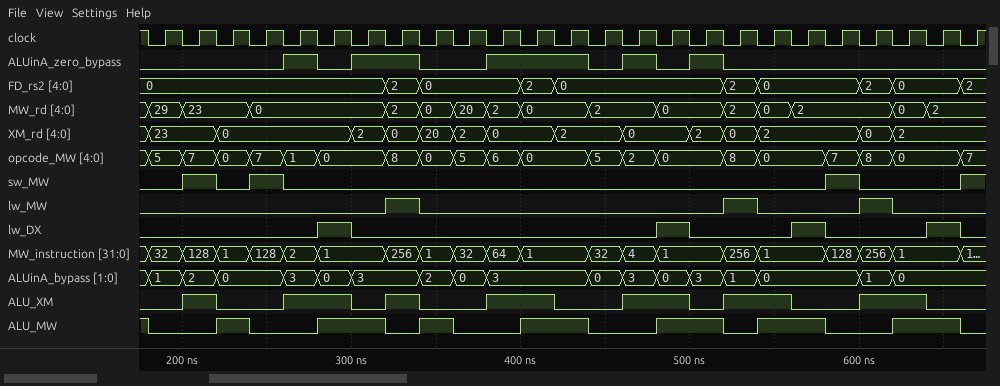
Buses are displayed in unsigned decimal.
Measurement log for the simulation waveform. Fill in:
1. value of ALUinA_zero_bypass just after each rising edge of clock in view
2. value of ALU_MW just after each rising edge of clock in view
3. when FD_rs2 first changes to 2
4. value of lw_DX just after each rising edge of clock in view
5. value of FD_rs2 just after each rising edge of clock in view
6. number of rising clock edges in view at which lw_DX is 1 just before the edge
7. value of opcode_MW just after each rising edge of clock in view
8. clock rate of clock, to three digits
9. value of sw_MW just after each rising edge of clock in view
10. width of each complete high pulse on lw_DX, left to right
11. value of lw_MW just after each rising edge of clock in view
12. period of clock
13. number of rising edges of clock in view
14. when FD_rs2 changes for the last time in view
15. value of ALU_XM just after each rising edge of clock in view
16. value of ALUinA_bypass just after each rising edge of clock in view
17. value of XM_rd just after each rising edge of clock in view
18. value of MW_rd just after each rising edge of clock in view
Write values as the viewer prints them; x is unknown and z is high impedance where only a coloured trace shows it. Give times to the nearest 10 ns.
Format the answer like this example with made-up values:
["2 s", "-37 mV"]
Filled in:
["0 0 0 0 1 0 1 1 0 0 1 1 1 0 1 0 1 0 0 0 0 0 0 0 0", "0 0 1 0 0 1 1 0 1 0 0 1 1 0 0 1 1 0 1 1 0 0 1 1 0", "320 ns", "0 0 0 0 0 1 0 0 0 0 0 0 0 0 0 1 0 0 0 1 0 0 0 1 0", "0, 0, 0, 0, 0, 0, 0, 2, 0, 0, 0, 2, 0, 0, 0, 0, 0, 2, 0, 0, 0, 2, 0, 0, 2", "4", "5, 7, 0, 7, 1, 0, 0, 8, 0, 5, 6, 0, 0, 5, 2, 0, 0, 8, 0, 0, 7, 8, 0, 0, 7", "50.0 MHz", "0 1 0 1 0 0 0 0 0 0 0 0 0 0 0 0 0 0 0 0 1 0 0 0 1", "20 ns, 20 ns, 20 ns, 20 ns", "0 0 0 0 0 0 0 1 0 0 0 0 0 0 0 0 0 1 0 0 0 1 0 0 0", "20 ns", "25", "660 ns", "0 1 0 0 1 1 0 1 0 0 1 1 0 0 1 1 0 1 1 0 0 1 1 0 0", "1, 2, 0, 0, 3, 0, 3, 3, 2, 0, 3, 3, 3, 0, 3, 0, 3, 1, 0, 0, 0, 1, 0, 0, 0", "23, 23, 0, 0, 0, 0, 2, 0, 20, 2, 0, 0, 2, 2, 0, 0, 2, 0, 2, 2, 2, 0, 2, 2, 2", "29, 23, 23, 0, 0, 0, 0, 2, 0, 20, 2, 0, 0, 2, 2, 0, 0, 2, 0, 2, 2, 2, 0, 2, 2"]
